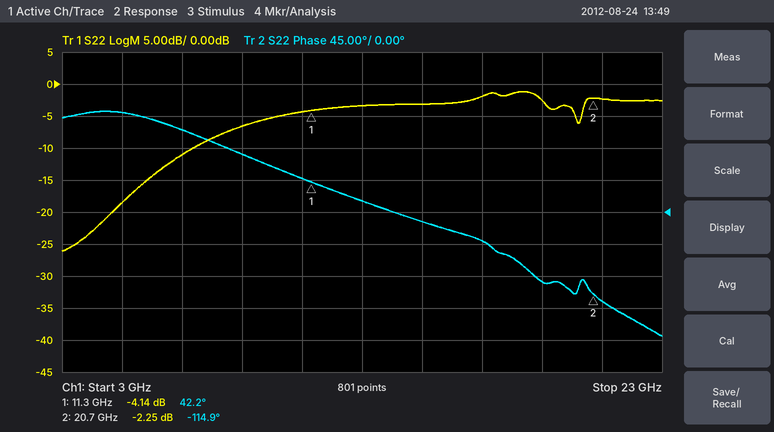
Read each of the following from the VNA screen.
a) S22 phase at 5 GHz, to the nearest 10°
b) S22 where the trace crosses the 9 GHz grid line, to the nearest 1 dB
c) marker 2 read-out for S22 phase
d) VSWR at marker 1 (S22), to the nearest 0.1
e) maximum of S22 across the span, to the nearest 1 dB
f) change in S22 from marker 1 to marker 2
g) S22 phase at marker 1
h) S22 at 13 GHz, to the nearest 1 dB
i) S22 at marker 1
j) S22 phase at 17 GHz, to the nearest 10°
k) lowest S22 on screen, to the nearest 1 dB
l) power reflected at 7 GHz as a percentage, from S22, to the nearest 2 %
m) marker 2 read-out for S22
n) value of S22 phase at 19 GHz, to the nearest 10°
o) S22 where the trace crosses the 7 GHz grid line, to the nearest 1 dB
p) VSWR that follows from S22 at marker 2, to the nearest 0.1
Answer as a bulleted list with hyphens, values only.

- 140°
- -7 dB
- -114.9°
- 4.3
- -1 dB
- 1.89 dB
- 42.2°
- -3 dB
- -4.14 dB
- -40°
- -26 dB
- 8 %
- -2.25 dB
- -100°
- -11 dB
- 7.8
